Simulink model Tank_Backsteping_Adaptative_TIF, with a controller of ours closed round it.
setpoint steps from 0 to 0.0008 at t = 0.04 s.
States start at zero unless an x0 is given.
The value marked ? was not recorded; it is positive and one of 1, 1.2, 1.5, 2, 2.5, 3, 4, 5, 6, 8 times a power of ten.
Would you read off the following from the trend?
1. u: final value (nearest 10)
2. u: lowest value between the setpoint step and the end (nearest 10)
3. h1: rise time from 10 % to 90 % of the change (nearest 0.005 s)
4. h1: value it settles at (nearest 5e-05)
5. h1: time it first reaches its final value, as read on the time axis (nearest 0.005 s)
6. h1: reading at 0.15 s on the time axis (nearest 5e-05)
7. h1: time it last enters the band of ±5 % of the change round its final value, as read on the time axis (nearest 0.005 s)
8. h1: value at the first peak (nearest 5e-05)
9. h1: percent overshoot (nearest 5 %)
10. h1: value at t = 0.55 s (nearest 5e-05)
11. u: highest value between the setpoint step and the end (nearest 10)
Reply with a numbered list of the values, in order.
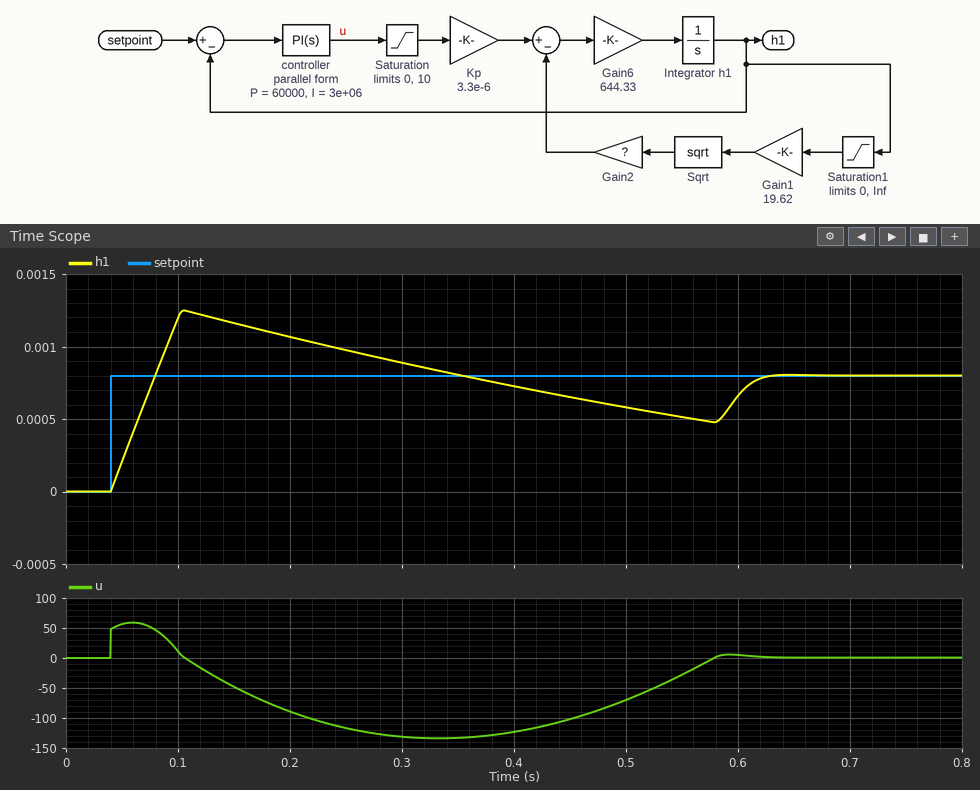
1. 0
2. -130
3. 0.030 s
4. 0.00080
5. 0.080 s
6. 0.00115
7. 0.615 s
8. 0.00125
9. 55 %
10. 0.00050
11. 60
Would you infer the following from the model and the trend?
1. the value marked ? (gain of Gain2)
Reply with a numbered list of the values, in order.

1. 2e-05
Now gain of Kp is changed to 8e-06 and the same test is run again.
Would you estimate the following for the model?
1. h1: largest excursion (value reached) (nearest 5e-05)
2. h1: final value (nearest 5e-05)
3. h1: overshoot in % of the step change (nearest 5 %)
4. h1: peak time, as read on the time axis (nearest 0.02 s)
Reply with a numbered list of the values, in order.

1. 0.00105
2. 0.00080
3. 30 %
4. 0.06 s
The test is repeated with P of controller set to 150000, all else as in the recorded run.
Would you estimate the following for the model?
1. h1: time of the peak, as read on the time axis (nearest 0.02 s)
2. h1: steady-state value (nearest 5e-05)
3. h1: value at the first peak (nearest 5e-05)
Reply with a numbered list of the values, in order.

1. 0.10 s
2. 0.00080
3. 0.00105
